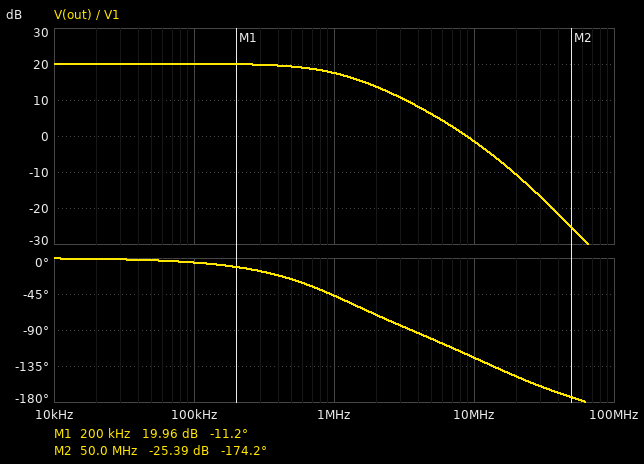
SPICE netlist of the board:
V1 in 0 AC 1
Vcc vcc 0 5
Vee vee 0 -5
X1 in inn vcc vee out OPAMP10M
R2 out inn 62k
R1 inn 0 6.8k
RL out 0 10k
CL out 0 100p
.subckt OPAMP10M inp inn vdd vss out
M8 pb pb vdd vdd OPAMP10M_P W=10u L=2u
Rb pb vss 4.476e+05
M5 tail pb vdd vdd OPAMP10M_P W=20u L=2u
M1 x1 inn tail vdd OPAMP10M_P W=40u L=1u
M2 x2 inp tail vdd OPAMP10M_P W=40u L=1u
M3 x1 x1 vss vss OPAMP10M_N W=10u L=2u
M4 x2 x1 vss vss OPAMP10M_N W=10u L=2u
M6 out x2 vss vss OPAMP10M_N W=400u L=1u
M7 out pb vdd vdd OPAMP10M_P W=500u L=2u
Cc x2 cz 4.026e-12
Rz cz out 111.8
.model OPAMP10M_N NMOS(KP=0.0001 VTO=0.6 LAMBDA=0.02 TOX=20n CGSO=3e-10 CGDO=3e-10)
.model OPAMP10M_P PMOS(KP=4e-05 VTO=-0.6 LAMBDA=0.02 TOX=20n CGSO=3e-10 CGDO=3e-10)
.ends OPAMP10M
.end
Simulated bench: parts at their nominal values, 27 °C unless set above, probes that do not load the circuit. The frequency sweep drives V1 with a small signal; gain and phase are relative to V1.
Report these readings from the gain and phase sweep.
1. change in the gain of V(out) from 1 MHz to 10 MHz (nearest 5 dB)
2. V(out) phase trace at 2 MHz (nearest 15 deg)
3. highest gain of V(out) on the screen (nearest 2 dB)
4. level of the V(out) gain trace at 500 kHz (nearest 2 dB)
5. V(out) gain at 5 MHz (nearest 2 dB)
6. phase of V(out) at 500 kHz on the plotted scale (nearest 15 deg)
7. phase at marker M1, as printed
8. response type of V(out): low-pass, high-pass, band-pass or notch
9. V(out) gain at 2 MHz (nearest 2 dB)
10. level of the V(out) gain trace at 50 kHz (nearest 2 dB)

-20 dB
-75 deg
20 dB
20 dB
6 dB
-30 deg
-11.2 deg
low-pass
14 dB
20 dB
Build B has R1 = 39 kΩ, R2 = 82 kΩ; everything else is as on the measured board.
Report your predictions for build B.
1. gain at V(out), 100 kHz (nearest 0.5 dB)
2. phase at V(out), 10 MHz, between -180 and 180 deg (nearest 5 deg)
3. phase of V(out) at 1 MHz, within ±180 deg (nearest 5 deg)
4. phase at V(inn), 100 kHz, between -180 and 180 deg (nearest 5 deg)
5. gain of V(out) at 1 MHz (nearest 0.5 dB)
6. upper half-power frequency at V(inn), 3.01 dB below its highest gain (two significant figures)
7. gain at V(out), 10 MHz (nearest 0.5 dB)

10.0 dB
-120 deg
-15 deg
0 deg
9.5 dB
4.2 MHz
-0.5 dB
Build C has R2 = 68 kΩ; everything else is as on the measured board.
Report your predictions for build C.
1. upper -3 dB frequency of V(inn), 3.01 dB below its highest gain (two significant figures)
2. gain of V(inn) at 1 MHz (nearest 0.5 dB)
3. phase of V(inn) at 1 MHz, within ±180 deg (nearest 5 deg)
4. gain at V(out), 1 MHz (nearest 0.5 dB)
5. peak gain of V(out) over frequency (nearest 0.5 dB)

1.0 MHz
-3.0 dB
-50 deg
18.0 dB
21.0 dB
